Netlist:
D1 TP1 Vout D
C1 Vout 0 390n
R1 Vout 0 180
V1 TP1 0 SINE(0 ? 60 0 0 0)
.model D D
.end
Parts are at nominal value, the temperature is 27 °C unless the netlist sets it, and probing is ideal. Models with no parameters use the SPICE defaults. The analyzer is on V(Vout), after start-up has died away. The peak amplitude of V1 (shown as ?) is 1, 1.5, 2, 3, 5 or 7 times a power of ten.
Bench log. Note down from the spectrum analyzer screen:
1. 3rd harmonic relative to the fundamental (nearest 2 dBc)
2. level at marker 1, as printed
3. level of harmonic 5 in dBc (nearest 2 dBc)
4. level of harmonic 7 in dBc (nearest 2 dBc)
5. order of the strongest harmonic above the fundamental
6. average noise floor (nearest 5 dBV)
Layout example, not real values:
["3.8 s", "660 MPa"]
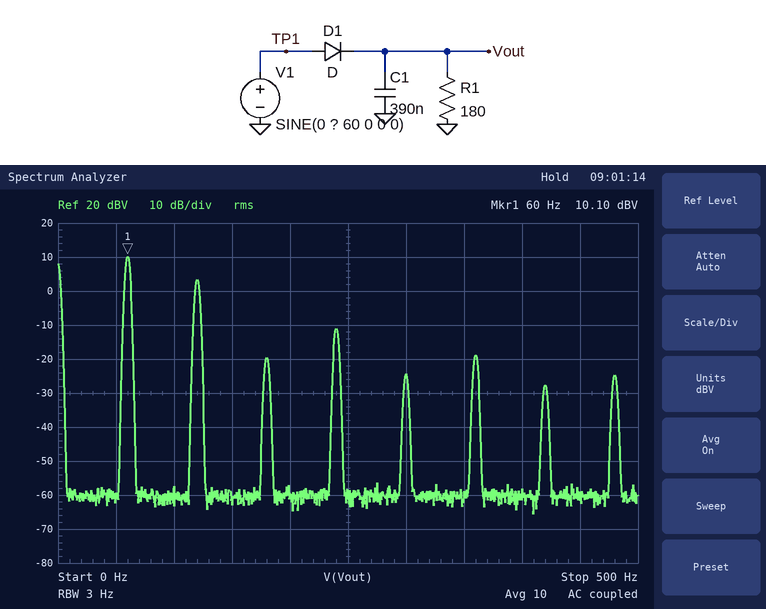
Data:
["-30 dBc", "10.10 dBV", "-34 dBc", "-38 dBc", "2", "-60 dBV"]
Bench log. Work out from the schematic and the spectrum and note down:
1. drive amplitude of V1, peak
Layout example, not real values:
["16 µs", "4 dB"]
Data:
["10 V"]
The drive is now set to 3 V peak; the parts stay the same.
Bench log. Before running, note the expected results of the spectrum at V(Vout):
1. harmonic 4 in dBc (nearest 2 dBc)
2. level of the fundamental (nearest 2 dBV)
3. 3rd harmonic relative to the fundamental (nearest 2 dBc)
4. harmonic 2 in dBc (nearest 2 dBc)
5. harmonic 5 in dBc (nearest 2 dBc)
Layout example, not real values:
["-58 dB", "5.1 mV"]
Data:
["-22 dBc", "-2 dBV", "-18 dBc", "-6 dBc", "-24 dBc"]
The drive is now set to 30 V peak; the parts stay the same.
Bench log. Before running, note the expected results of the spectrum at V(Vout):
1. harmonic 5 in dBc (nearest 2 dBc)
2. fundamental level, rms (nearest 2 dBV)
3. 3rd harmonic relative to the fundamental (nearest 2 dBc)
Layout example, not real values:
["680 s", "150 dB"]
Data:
["-44 dBc", "20 dBV", "-40 dBc"]
